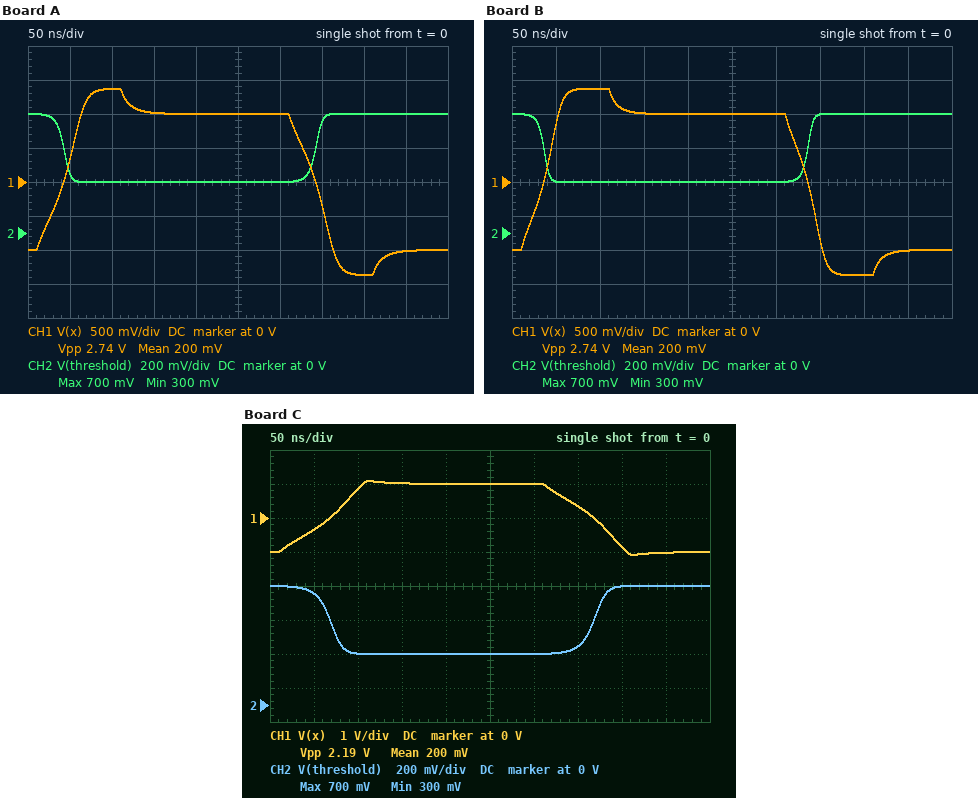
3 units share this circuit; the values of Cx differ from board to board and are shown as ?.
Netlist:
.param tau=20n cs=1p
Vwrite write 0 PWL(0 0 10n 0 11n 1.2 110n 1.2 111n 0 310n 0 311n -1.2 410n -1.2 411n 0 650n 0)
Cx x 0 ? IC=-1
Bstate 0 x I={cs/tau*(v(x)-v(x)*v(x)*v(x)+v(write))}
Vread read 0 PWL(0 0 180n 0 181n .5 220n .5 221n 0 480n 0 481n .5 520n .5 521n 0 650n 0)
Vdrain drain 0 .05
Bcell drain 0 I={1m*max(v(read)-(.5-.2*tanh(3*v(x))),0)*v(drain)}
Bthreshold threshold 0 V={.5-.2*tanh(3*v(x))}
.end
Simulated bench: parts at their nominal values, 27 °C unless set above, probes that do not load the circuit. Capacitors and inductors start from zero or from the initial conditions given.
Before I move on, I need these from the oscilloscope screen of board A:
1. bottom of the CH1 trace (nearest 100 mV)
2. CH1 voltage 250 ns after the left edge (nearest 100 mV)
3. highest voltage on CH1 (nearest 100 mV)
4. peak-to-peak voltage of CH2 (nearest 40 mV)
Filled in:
-1.4 V
1.0 V
1.4 V
400 mV
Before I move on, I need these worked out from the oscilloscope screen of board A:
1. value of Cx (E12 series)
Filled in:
1.5 pF
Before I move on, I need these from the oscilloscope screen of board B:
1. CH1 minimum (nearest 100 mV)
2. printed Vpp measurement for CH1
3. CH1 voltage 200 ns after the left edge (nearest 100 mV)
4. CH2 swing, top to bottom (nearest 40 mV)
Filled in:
-1.4 V
2.74 V
1.0 V
400 mV
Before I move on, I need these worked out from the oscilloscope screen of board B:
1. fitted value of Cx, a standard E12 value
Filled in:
1.2 pF
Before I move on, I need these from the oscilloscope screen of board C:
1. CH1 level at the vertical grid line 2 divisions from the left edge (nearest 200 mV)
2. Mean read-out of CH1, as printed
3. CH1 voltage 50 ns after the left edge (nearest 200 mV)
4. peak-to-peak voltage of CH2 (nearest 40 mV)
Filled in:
800 mV
200 mV
-400 mV
400 mV
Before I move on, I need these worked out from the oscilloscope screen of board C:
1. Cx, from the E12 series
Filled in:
2.7 pF
